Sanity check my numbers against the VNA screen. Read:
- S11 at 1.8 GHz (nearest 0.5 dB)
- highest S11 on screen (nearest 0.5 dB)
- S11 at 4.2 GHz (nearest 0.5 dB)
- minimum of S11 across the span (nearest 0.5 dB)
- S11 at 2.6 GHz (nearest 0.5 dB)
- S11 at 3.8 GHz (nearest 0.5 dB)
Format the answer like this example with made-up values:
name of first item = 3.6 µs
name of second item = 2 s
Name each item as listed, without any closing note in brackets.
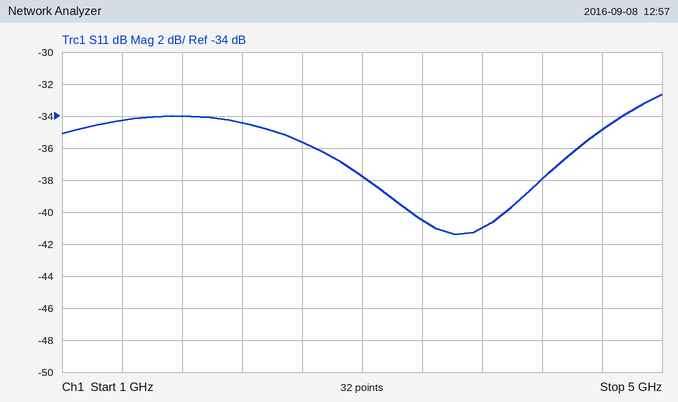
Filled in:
S11 at 1.8 GHz = -34.0 dB
highest S11 on screen = -32.5 dB
S11 at 4.2 GHz = -38.0 dB
minimum of S11 across the span = -41.5 dB
S11 at 2.6 GHz = -35.5 dB
S11 at 3.8 GHz = -41.0 dB
